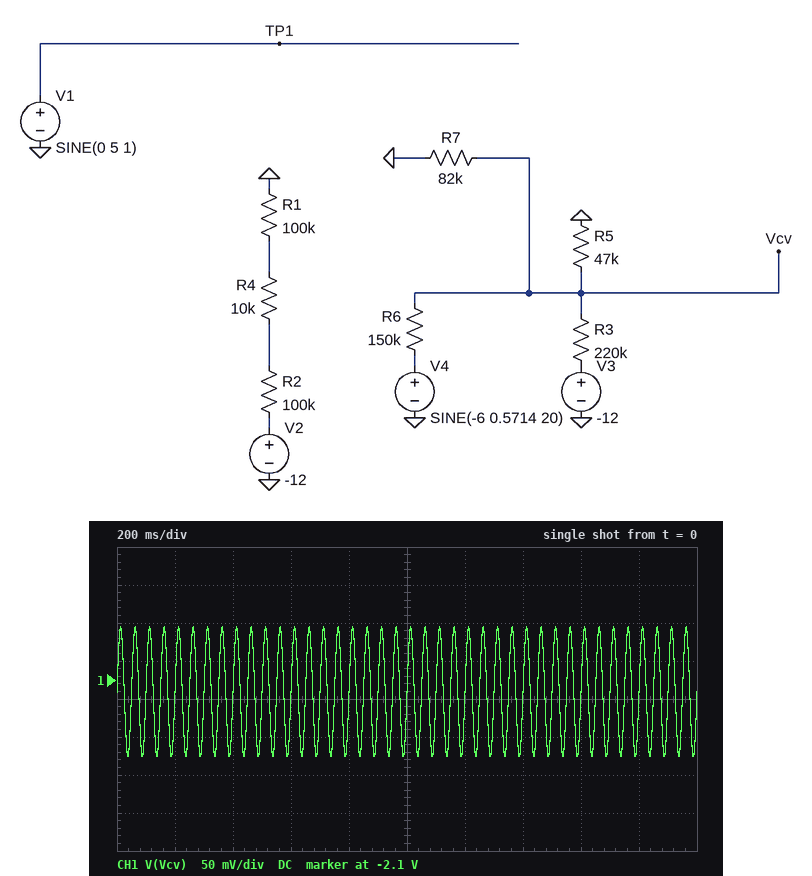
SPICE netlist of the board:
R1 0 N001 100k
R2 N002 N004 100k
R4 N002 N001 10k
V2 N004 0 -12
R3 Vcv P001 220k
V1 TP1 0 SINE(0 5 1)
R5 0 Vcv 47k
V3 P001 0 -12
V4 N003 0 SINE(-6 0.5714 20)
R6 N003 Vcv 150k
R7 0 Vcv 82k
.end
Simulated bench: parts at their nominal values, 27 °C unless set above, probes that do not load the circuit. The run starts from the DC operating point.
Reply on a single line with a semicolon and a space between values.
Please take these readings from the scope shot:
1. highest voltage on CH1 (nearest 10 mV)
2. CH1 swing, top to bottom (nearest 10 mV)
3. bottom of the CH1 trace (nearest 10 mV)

-2.03 V; 170 mV; -2.20 V
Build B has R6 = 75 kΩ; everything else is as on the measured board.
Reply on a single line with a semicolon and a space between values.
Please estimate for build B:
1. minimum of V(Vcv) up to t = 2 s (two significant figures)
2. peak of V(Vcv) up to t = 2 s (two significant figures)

-2.8 V; -2.5 V
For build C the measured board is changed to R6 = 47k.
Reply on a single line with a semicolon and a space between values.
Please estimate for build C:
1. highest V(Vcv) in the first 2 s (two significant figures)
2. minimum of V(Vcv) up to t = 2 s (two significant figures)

-2.9 V; -3.3 V
